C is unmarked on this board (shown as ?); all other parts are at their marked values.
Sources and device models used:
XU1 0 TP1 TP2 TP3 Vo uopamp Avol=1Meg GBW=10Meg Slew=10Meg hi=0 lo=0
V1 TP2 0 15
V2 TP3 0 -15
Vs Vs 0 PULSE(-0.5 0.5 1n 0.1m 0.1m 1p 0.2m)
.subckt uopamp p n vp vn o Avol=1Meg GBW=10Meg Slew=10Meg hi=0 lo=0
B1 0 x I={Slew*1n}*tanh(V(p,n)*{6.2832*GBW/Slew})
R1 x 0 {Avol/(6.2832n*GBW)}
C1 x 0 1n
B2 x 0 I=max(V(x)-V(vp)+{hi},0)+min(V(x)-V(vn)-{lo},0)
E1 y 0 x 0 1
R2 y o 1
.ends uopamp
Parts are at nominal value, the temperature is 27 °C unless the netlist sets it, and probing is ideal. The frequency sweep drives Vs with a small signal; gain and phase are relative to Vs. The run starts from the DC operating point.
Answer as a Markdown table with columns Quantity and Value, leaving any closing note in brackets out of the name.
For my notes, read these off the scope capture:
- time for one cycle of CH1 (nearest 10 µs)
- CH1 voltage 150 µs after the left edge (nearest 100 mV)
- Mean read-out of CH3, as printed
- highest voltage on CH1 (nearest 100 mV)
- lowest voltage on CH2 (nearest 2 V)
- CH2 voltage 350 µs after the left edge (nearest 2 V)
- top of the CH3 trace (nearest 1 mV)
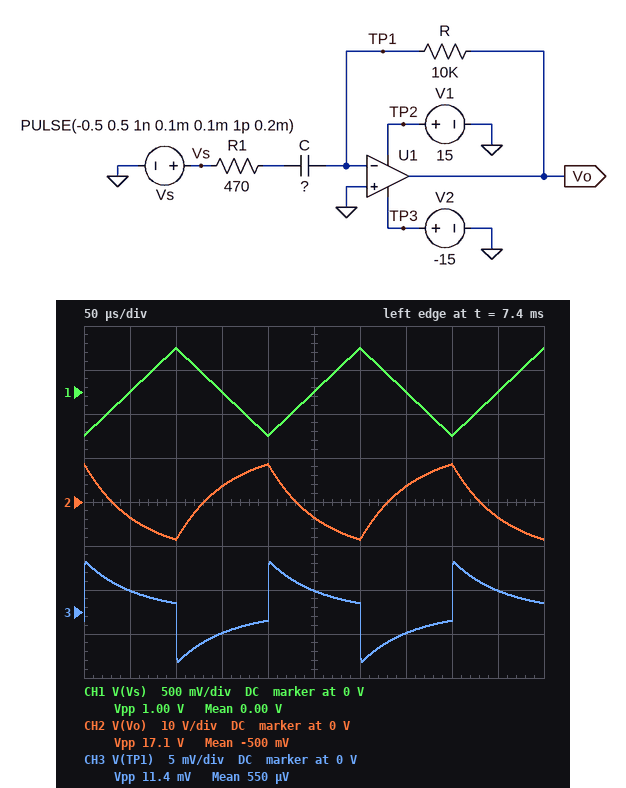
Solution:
| Quantity | Value |
|---|---|
| time for one cycle of CH1 | 200 µs |
| CH1 voltage 150 µs after the left edge | 0 V |
| Mean read-out of CH3, as printed | 550 µV |
| highest voltage on CH1 | 500 mV |
| lowest voltage on CH2 | -8 V |
| CH2 voltage 350 µs after the left edge | 4 V |
| top of the CH3 trace | 6 mV |
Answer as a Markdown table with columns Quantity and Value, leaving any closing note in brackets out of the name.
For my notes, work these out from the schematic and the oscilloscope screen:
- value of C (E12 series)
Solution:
| Quantity | Value |
|---|---|
| value of C | 120 nF |
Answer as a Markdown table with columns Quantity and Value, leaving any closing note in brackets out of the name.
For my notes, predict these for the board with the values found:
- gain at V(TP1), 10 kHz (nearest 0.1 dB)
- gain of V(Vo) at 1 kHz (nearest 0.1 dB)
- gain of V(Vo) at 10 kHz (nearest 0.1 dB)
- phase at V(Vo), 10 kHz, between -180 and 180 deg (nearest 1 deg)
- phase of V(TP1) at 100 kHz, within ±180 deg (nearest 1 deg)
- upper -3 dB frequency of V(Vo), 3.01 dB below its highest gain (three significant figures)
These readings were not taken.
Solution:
| Quantity | Value |
|---|---|
| gain at V(TP1), 10 kHz | -33.7 dB |
| gain of V(Vo) at 1 kHz | 17.0 dB |
| gain of V(Vo) at 10 kHz | 26.3 dB |
| phase at V(Vo), 10 kHz, between -180 and 180 deg | -165 deg |
| phase of V(TP1) at 100 kHz, within ±180 deg | 79 deg |
| upper -3 dB frequency of V(Vo), 3.01 dB below its highest gain | 452 kHz |
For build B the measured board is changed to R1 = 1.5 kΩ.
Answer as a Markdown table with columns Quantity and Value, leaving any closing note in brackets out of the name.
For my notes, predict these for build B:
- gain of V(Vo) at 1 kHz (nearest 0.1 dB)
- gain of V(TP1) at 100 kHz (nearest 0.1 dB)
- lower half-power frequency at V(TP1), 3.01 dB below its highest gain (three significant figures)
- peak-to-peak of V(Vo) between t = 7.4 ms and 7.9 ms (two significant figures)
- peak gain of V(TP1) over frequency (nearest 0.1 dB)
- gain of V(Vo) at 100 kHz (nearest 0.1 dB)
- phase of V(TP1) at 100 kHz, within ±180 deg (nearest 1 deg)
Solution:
| Quantity | Value |
|---|---|
| gain of V(Vo) at 1 kHz | 14.0 dB |
| gain of V(TP1) at 100 kHz | -23.5 dB |
| lower half-power frequency at V(TP1), 3.01 dB below its highest gain | 1.30 MHz |
| peak-to-peak of V(Vo) between t = 7.4 ms and 7.9 ms | 6.5 V |
| peak gain of V(TP1) over frequency | -1.2 dB |
| gain of V(Vo) at 100 kHz | 16.5 dB |
| phase of V(TP1) at 100 kHz, within ±180 deg | 86 deg |
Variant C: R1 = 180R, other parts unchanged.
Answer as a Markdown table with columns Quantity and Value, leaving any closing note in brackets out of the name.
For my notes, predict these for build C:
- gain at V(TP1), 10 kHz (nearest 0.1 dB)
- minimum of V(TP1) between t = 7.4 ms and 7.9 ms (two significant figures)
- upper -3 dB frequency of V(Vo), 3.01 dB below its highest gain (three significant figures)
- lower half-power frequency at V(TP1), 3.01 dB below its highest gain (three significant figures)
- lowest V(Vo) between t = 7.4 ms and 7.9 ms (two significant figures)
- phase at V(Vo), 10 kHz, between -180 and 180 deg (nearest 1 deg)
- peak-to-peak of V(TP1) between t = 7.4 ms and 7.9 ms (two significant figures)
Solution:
| Quantity | Value |
|---|---|
| gain at V(TP1), 10 kHz | -26.8 dB |
| minimum of V(TP1) between t = 7.4 ms and 7.9 ms | -16 mV |
| upper -3 dB frequency of V(Vo), 3.01 dB below its highest gain | 184 kHz |
| lower half-power frequency at V(TP1), 3.01 dB below its highest gain | 170 kHz |
| lowest V(Vo) between t = 7.4 ms and 7.9 ms | -12 V |
| phase at V(Vo), 10 kHz, between -180 and 180 deg | -146 deg |
| peak-to-peak of V(TP1) between t = 7.4 ms and 7.9 ms | 32 mV |
